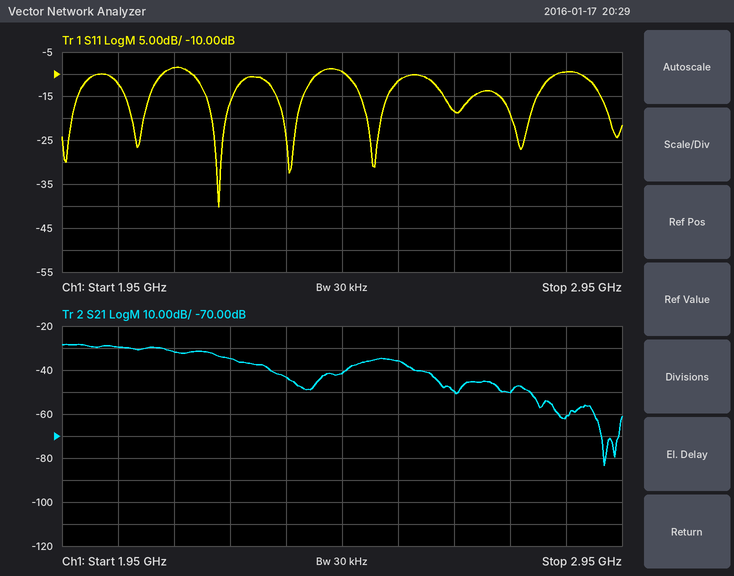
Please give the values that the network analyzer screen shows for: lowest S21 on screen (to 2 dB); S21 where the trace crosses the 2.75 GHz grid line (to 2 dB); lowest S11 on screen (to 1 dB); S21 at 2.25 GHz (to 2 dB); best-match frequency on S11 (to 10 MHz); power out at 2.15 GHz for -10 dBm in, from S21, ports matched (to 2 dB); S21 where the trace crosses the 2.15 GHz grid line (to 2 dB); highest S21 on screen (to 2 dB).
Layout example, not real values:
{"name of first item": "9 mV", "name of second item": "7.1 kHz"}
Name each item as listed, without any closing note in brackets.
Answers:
{"lowest S21 on screen": "-84 dB", "S21 where the trace crosses the 2.75 GHz grid line": "-50 dB", "lowest S11 on screen": "-40 dB", "S21 at 2.25 GHz": "-34 dB", "best-match frequency on S11": "2.23 GHz", "power out at 2.15 GHz for -10 dBm in, from S21, ports matched": "-42 dBm", "S21 where the trace crosses the 2.15 GHz grid line": "-32 dB", "highest S21 on screen": "-28 dB"}
